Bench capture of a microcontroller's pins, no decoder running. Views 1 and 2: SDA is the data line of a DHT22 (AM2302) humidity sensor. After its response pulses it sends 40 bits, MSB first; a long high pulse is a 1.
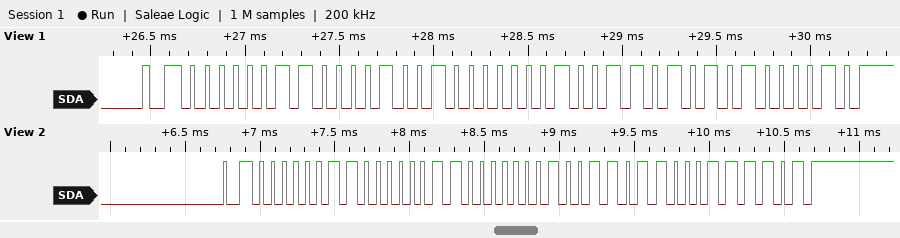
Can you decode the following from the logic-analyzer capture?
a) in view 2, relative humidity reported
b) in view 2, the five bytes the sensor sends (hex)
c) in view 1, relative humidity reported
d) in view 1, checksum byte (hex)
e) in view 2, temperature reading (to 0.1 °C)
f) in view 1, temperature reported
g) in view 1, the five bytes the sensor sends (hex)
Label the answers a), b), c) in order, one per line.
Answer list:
a) 77.1 %
b) 03 03 01 36 3D
c) 77.7 %
d) 0x42
e) 31.0 °C
f) 30.9 °C
g) 03 09 01 35 42
